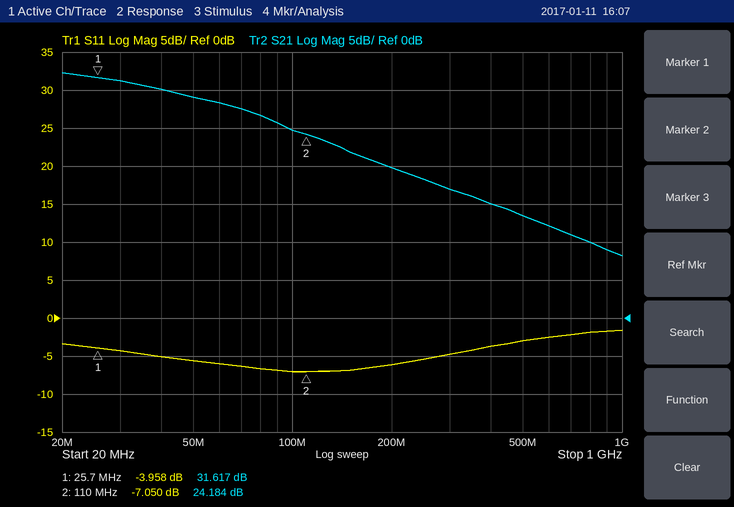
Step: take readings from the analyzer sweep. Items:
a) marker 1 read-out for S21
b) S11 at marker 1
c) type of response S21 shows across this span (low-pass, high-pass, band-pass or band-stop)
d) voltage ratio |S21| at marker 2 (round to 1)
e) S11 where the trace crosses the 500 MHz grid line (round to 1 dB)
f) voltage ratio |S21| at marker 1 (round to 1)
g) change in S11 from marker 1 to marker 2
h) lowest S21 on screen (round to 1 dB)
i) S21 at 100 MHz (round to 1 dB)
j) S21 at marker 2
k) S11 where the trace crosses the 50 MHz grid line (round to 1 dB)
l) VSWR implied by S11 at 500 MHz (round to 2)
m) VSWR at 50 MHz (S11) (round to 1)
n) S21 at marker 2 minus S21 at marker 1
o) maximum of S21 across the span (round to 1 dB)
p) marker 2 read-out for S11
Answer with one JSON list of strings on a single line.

["31.617 dB", "-3.958 dB", "low-pass", "16", "-3 dB", "38", "-3.092 dB", "8 dB", "25 dB", "24.184 dB", "-6 dB", "6", "3", "-7.433 dB", "32 dB", "-7.050 dB"]
